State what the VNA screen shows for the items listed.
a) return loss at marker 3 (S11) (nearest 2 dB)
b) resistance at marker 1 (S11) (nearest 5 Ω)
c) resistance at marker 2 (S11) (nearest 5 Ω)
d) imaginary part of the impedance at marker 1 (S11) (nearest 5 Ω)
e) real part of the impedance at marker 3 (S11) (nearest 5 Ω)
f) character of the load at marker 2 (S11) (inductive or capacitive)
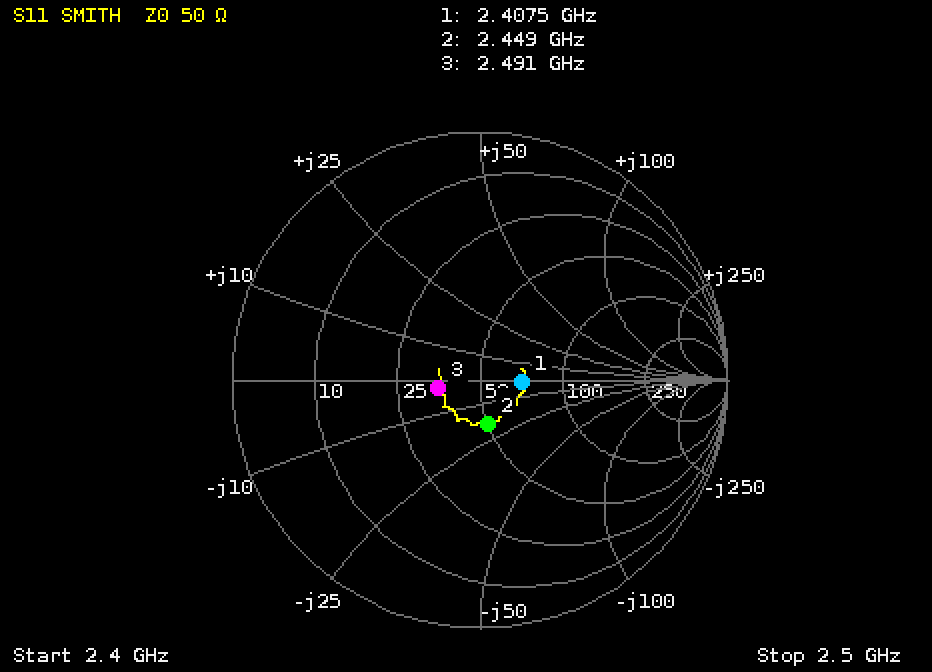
16 dB
70 Ω
50 Ω
0 Ω
35 Ω
capacitive
